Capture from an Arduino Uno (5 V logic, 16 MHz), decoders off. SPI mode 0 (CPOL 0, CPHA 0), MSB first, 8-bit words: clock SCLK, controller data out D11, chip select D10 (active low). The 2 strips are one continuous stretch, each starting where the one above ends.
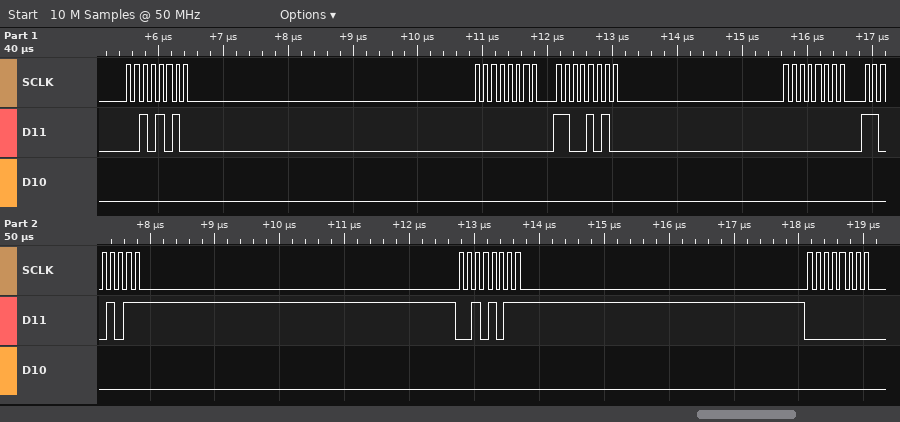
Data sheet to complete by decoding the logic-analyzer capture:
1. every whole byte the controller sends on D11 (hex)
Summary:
2A 00 CA 00 CB 2B 00
